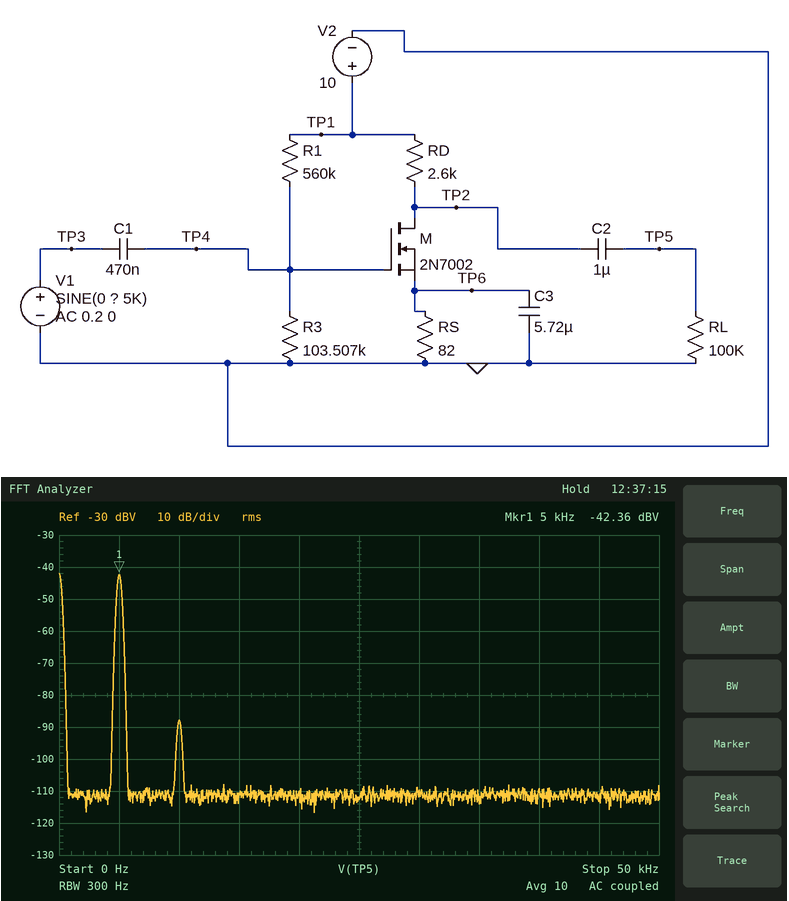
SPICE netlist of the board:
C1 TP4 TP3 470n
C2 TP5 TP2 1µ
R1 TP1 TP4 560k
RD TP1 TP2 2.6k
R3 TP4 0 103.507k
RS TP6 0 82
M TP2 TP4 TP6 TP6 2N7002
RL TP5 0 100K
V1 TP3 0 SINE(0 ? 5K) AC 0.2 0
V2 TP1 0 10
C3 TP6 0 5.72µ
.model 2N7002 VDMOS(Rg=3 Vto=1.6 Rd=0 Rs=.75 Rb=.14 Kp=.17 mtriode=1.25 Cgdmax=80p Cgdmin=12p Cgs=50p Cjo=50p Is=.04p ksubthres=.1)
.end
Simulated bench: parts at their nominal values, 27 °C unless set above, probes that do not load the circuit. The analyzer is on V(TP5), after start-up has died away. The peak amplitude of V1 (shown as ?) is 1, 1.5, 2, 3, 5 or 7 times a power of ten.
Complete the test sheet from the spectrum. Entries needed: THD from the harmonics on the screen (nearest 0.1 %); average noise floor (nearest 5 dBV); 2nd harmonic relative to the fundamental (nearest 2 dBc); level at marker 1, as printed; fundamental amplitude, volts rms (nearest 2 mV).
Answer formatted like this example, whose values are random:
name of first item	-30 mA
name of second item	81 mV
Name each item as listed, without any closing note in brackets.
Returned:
THD from the harmonics on the screen	0.5 %
average noise floor	-110 dBV
2nd harmonic relative to the fundamental	-46 dBc
level at marker 1, as printed	-42.36 dBV
fundamental amplitude, volts rms	8 mV
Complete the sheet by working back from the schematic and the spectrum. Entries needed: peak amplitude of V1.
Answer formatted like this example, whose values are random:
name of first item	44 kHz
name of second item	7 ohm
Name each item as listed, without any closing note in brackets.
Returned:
peak amplitude of V1	1.5 mV
